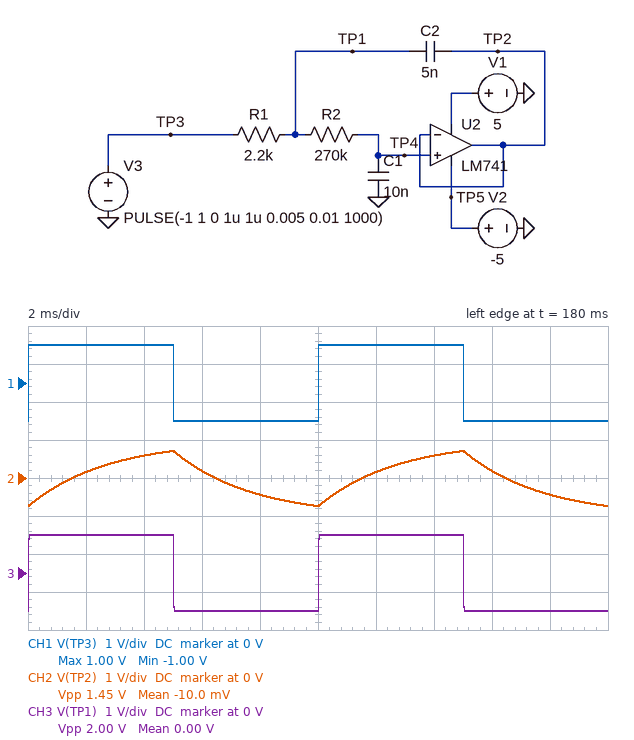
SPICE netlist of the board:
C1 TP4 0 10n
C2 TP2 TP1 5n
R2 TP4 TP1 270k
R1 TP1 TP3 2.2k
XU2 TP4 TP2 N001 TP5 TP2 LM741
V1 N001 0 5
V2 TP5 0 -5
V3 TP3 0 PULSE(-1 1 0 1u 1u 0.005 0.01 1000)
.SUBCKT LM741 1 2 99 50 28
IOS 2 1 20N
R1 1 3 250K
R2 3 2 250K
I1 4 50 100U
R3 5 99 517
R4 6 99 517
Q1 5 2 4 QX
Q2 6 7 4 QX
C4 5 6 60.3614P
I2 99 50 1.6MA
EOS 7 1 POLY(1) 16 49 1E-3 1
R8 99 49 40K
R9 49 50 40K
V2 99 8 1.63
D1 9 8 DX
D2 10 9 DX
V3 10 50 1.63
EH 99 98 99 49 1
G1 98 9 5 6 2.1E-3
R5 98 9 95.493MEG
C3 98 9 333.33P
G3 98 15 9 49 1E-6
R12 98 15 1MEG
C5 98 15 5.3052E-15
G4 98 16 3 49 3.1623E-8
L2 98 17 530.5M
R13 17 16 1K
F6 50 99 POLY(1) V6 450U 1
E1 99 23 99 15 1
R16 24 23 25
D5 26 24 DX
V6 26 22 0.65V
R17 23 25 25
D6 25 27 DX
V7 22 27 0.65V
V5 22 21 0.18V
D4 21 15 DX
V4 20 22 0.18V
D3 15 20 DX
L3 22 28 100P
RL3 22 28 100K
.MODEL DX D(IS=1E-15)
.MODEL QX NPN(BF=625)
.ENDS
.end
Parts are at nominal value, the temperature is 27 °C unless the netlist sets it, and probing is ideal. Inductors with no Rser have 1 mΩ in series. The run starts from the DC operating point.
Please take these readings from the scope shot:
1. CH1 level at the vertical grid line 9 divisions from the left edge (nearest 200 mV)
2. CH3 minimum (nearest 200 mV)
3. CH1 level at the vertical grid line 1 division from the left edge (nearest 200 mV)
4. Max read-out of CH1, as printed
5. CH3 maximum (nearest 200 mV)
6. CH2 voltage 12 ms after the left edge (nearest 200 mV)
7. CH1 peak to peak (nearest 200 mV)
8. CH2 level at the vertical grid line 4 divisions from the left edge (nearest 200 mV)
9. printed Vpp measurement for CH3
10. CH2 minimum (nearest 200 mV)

-1.0 V
-1.0 V
1.0 V
1.00 V
1.0 V
200 mV
2.0 V
-400 mV
2.00 V
-800 mV
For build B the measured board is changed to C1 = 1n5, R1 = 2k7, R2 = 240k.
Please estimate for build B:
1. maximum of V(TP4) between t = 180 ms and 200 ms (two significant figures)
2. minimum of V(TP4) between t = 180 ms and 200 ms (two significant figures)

990 mV
-1.0 V
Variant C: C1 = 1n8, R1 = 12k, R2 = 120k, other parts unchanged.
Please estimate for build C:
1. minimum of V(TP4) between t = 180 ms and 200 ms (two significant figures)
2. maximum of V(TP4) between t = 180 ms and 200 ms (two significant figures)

-1.0 V
990 mV
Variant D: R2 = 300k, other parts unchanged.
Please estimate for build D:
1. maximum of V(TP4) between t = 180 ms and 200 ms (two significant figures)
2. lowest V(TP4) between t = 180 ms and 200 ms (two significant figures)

660 mV
-700 mV
